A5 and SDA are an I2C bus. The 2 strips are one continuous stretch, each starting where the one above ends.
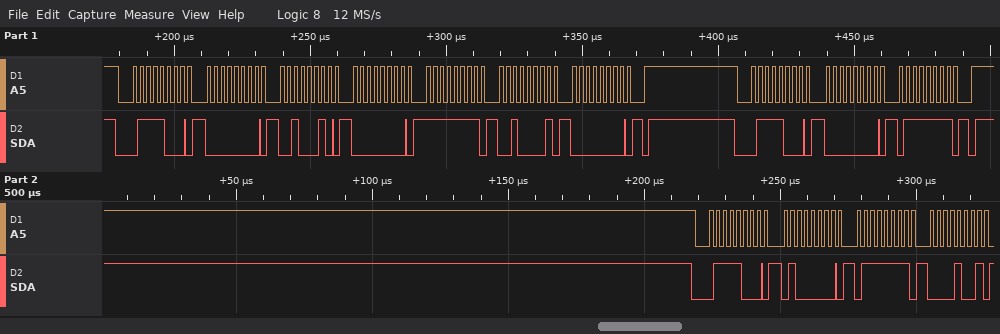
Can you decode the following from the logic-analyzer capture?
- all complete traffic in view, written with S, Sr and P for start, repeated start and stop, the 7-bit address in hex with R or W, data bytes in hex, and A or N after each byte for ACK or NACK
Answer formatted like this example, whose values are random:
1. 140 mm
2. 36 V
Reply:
1. S 3CW A 00 A 22 A 00 A FF A 21 A 00 A P S 3CW A 00 A 7F A P S 3CW A 40 A 7F A 09 A
